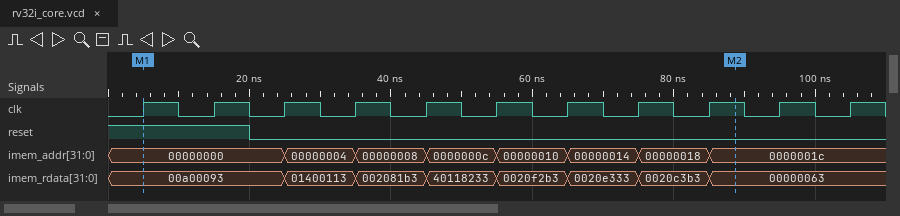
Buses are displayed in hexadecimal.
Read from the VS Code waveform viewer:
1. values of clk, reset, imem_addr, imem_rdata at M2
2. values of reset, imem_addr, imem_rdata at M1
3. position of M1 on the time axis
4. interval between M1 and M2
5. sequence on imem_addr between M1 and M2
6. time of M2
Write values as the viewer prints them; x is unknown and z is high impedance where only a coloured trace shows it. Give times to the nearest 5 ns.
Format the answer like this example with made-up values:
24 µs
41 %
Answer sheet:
clk=1, reset=0, imem_addr=0000001c, imem_rdata=00000063
reset=1, imem_addr=00000000, imem_rdata=00a00093
5 ns
85 ns
00000000, 00000004, 00000008, 0000000c, 00000010, 00000014, 00000018, 0000001c
90 ns
